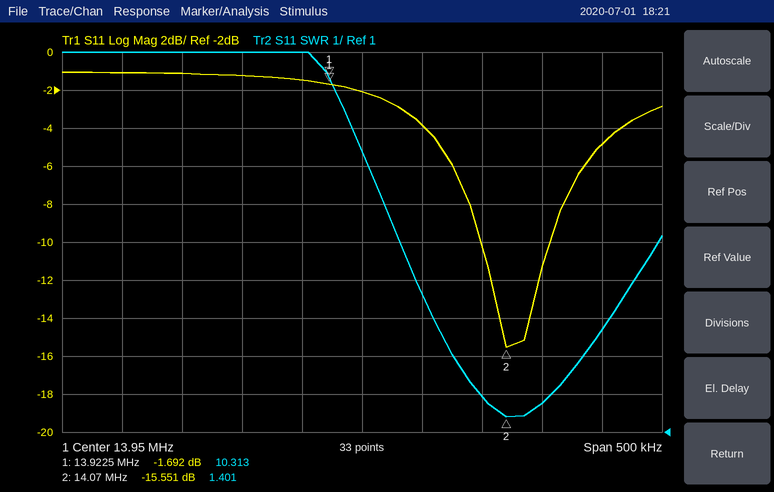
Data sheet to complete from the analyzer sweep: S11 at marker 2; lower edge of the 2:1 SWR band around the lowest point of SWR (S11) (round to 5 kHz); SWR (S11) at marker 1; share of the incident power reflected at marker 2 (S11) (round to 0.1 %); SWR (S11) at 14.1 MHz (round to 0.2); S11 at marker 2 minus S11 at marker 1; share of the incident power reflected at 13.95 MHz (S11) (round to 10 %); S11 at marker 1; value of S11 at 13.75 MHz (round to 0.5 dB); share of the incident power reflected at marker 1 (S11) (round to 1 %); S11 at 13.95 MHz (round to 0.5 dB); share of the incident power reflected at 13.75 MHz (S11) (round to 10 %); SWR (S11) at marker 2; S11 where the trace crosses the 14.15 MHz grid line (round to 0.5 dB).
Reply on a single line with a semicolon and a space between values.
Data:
-15.551 dB; 14.050 MHz; 10.313; 2.8 %; 1.8; -13.859 dB; 60 %; -1.692 dB; -1.0 dB; 68 %; -2.0 dB; 80 %; 1.401; -5.0 dB
